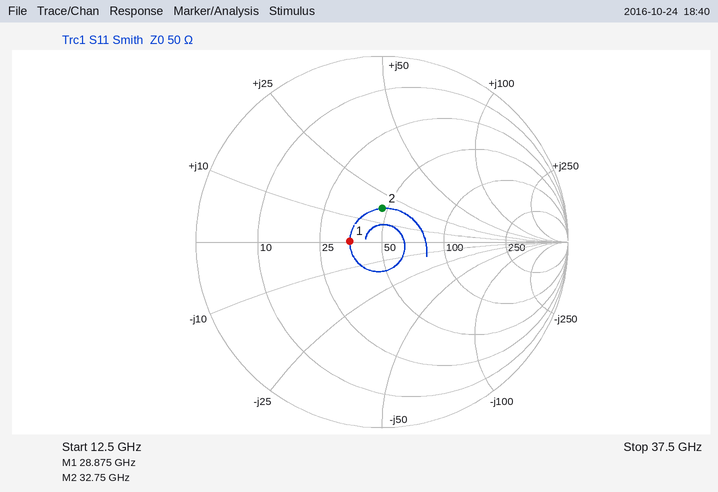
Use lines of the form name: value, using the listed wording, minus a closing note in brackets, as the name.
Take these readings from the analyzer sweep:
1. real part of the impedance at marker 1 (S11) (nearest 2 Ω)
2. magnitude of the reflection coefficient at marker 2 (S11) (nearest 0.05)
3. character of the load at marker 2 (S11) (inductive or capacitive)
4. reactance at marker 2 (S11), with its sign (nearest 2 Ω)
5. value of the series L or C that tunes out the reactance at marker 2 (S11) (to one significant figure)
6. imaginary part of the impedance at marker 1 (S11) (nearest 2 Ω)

real part of the impedance at marker 1 (S11): 36 Ω
magnitude of the reflection coefficient at marker 2 (S11): 0.20
character of the load at marker 2 (S11): inductive
reactance at marker 2 (S11), with its sign: +18 Ω
value of the series L or C that tunes out the reactance at marker 2 (S11): 300 fF
imaginary part of the impedance at marker 1 (S11): 0 Ω
